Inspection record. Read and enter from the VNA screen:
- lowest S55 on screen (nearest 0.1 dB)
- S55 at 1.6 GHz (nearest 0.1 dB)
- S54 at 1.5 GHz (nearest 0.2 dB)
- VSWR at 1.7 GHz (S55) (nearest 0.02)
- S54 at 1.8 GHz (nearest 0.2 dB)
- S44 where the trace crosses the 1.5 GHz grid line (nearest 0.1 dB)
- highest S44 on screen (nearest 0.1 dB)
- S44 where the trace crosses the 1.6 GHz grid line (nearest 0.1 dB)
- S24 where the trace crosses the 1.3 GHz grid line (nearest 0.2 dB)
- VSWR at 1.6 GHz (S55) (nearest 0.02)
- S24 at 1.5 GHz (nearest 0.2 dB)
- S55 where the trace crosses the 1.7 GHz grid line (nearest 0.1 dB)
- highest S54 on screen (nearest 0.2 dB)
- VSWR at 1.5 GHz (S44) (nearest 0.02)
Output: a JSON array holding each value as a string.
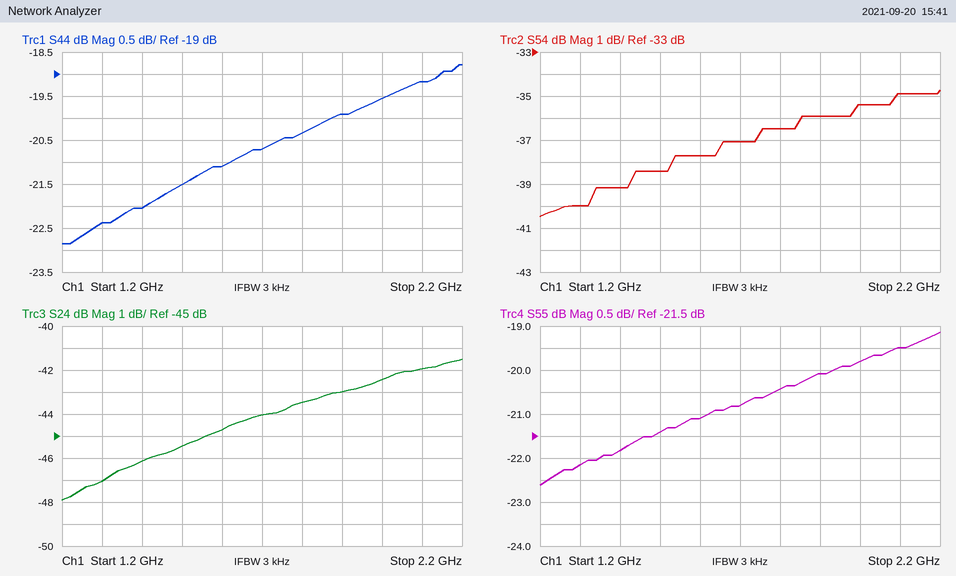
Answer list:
["-22.6 dB", "-21.1 dB", "-38.4 dB", "1.20", "-36.4 dB", "-21.5 dB", "-18.8 dB", "-21.1 dB", "-47.0 dB", "1.20", "-45.4 dB", "-20.8 dB", "-34.8 dB", "1.18"]
